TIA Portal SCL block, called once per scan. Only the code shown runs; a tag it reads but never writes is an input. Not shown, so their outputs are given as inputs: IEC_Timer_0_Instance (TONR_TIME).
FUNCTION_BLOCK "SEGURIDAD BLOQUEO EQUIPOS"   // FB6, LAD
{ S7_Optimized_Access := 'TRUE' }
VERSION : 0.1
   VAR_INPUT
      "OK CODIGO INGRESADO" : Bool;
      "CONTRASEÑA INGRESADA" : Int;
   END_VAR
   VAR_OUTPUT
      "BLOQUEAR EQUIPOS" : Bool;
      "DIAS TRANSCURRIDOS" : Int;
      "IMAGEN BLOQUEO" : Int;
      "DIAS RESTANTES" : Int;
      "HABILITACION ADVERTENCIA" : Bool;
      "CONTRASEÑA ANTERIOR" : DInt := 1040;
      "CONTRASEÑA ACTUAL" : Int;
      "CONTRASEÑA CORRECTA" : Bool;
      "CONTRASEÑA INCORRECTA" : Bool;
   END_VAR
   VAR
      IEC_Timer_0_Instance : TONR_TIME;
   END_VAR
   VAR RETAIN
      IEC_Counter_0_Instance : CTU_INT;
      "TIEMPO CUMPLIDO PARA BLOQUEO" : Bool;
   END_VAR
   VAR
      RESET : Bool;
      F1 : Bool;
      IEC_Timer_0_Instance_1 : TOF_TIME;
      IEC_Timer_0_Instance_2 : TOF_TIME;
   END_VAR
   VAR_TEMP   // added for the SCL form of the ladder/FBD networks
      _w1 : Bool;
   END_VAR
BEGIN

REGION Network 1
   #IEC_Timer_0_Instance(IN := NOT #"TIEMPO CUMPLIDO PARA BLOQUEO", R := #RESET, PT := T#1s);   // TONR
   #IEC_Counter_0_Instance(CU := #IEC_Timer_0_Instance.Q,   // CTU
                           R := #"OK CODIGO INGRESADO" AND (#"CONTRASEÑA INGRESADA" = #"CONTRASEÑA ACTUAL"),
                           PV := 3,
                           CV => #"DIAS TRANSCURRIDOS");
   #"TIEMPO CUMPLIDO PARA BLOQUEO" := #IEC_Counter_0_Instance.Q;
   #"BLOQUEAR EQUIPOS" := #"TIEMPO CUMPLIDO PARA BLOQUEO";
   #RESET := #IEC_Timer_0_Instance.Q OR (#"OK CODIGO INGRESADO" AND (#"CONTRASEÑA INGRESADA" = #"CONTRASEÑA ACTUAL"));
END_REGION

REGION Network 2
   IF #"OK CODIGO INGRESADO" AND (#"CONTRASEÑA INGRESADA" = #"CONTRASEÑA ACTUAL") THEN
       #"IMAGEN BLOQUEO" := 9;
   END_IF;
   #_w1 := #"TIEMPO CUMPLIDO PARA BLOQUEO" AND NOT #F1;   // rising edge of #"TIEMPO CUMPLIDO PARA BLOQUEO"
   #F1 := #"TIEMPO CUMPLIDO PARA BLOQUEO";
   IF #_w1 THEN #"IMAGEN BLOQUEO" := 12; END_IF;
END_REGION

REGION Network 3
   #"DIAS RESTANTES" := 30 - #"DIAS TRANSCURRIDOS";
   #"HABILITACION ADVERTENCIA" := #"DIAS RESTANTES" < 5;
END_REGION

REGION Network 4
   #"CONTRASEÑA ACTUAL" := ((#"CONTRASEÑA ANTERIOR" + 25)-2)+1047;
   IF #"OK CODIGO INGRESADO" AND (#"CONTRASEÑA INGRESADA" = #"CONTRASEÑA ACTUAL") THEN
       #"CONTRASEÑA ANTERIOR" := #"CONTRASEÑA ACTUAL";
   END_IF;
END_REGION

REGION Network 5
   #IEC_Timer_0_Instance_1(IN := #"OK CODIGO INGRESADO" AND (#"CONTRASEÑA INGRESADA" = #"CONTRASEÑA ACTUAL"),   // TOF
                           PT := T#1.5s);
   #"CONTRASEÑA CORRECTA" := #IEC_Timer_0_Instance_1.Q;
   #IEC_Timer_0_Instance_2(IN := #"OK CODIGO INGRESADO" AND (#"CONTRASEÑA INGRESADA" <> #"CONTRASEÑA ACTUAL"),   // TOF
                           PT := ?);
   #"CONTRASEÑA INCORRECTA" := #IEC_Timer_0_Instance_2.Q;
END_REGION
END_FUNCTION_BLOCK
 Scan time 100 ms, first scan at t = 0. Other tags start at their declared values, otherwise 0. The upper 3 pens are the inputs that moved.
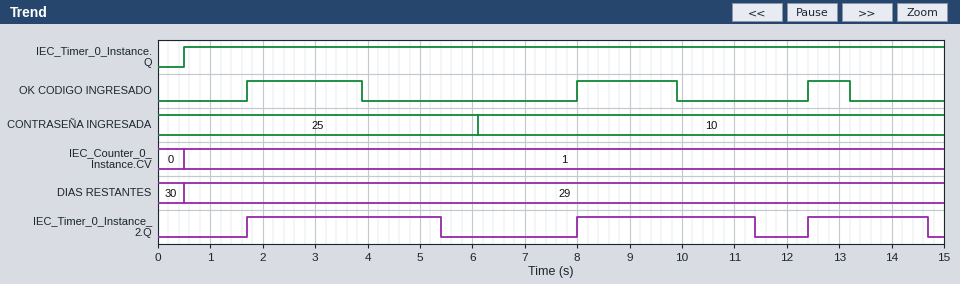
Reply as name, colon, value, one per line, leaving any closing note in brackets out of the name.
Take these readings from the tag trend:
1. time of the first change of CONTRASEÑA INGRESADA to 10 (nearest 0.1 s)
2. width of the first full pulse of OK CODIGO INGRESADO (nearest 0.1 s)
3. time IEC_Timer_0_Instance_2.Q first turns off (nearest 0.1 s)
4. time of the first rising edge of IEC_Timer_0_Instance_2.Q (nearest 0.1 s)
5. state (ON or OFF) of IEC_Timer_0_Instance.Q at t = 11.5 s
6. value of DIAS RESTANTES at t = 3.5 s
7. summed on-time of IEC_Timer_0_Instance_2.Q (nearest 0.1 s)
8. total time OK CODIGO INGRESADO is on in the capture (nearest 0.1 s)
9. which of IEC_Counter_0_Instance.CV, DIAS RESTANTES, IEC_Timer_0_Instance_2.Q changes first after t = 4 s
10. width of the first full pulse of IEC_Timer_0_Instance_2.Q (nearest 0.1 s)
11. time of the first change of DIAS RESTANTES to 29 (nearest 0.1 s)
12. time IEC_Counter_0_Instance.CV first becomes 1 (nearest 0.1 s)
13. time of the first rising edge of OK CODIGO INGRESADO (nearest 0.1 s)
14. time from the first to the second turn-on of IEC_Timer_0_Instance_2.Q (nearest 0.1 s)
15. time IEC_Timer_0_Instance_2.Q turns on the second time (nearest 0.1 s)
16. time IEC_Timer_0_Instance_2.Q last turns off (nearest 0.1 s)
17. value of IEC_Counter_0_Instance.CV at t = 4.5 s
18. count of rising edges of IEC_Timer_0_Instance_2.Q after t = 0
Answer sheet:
time of the first change of CONTRASEÑA INGRESADA to 10: 6.1 s
width of the first full pulse of OK CODIGO INGRESADO: 2.2 s
time IEC_Timer_0_Instance_2.Q first turns off: 5.4 s
time of the first rising edge of IEC_Timer_0_Instance_2.Q: 1.7 s
state (ON or OFF) of IEC_Timer_0_Instance.Q at t = 11.5 s: ON
value of DIAS RESTANTES at t = 3.5 s: 29
summed on-time of IEC_Timer_0_Instance_2.Q: 9.4 s
total time OK CODIGO INGRESADO is on in the capture: 4.9 s
which of IEC_Counter_0_Instance.CV, DIAS RESTANTES, IEC_Timer_0_Instance_2.Q changes first after t = 4 s: IEC_Timer_0_Instance_2.Q
width of the first full pulse of IEC_Timer_0_Instance_2.Q: 3.7 s
time of the first change of DIAS RESTANTES to 29: 0.5 s
time IEC_Counter_0_Instance.CV first becomes 1: 0.5 s
time of the first rising edge of OK CODIGO INGRESADO: 1.7 s
time from the first to the second turn-on of IEC_Timer_0_Instance_2.Q: 6.3 s
time IEC_Timer_0_Instance_2.Q turns on the second time: 8.0 s
time IEC_Timer_0_Instance_2.Q last turns off: 14.7 s
value of IEC_Counter_0_Instance.CV at t = 4.5 s: 1
count of rising edges of IEC_Timer_0_Instance_2.Q after t = 0: 3
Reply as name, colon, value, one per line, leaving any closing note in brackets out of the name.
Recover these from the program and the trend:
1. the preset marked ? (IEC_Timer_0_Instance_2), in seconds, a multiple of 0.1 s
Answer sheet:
the preset marked ? (IEC_Timer_0_Instance_2), in seconds, a multiple of 0.1 s: 1.5 s
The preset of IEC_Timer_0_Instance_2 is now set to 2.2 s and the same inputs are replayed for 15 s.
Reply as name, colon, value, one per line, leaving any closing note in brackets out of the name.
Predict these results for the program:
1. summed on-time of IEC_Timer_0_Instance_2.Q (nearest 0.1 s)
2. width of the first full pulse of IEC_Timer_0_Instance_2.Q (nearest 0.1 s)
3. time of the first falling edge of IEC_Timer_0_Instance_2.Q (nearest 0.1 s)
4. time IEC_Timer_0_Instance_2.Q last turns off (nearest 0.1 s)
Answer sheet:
summed on-time of IEC_Timer_0_Instance_2.Q: 11.1 s
width of the first full pulse of IEC_Timer_0_Instance_2.Q: 4.4 s
time of the first falling edge of IEC_Timer_0_Instance_2.Q: 6.1 s
time IEC_Timer_0_Instance_2.Q last turns off: 12.1 s
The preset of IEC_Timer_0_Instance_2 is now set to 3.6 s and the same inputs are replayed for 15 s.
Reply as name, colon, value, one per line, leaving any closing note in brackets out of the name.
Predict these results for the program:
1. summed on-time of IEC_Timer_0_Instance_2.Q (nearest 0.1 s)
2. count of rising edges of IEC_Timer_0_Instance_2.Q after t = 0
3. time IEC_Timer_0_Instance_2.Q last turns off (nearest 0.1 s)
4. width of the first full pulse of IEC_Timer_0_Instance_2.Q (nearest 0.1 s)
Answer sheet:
summed on-time of IEC_Timer_0_Instance_2.Q: 12.8 s
count of rising edges of IEC_Timer_0_Instance_2.Q after t = 0: 2
time IEC_Timer_0_Instance_2.Q last turns off: 7.5 s
width of the first full pulse of IEC_Timer_0_Instance_2.Q: 5.8 s
